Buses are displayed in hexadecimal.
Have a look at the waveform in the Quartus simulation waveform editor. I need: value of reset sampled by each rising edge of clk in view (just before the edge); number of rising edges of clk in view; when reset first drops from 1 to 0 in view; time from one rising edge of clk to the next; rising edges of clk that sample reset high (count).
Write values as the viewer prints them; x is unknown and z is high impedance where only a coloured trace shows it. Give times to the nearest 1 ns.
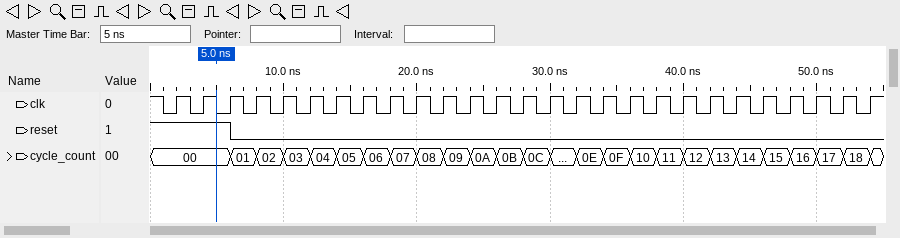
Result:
1 1 1 0 0 0 0 0 0 0 0 0 0 0 0 0 0 0 0 0 0 0 0 0 0 0 0
27
6 ns
2 ns
3
